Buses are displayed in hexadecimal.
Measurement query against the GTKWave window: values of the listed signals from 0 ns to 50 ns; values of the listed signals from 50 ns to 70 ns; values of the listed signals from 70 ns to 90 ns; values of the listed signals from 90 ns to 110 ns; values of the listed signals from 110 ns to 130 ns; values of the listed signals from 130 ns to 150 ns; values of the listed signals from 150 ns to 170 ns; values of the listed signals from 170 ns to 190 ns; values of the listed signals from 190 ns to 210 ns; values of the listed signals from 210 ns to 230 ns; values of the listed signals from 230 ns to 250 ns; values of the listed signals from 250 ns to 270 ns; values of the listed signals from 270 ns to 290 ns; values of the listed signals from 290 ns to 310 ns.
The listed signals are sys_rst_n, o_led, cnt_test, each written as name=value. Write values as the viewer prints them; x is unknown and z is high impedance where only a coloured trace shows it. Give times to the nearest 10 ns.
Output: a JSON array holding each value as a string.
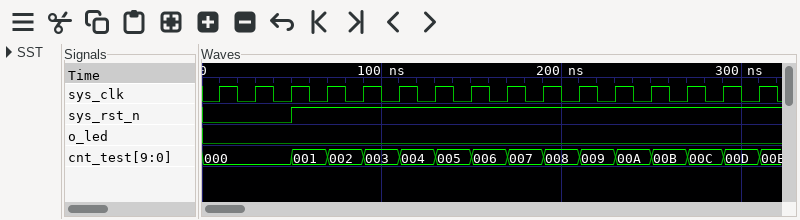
["sys_rst_n=0, o_led=0, cnt_test=000", "sys_rst_n=1, o_led=0, cnt_test=001", "sys_rst_n=1, o_led=0, cnt_test=002", "sys_rst_n=1, o_led=0, cnt_test=003", "sys_rst_n=1, o_led=0, cnt_test=004", "sys_rst_n=1, o_led=0, cnt_test=005", "sys_rst_n=1, o_led=0, cnt_test=006", "sys_rst_n=1, o_led=0, cnt_test=007", "sys_rst_n=1, o_led=0, cnt_test=008", "sys_rst_n=1, o_led=0, cnt_test=009", "sys_rst_n=1, o_led=0, cnt_test=00A", "sys_rst_n=1, o_led=0, cnt_test=00B", "sys_rst_n=1, o_led=0, cnt_test=00C", "sys_rst_n=1, o_led=0, cnt_test=00D"]
